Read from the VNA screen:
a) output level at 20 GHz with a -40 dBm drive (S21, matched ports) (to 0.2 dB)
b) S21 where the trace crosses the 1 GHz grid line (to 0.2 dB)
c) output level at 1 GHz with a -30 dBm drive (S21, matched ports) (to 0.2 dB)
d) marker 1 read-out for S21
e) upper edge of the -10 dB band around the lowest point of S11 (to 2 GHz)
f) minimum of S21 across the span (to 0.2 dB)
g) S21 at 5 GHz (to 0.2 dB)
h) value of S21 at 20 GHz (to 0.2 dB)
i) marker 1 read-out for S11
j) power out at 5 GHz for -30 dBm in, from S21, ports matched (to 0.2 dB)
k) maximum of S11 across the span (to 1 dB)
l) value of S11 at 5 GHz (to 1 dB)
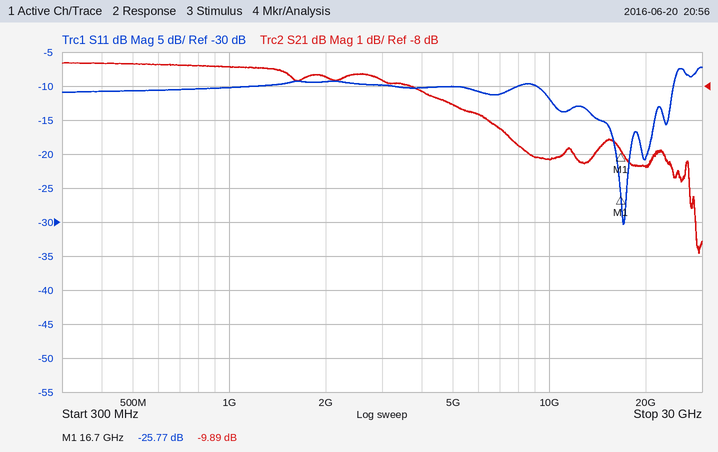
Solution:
-50.4 dBm
-7.4 dB
-37.4 dBm
-9.89 dB
24 GHz
-13.0 dB
-8.6 dB
-10.4 dB
-25.77 dB
-38.6 dBm
-7 dB
-10 dB
